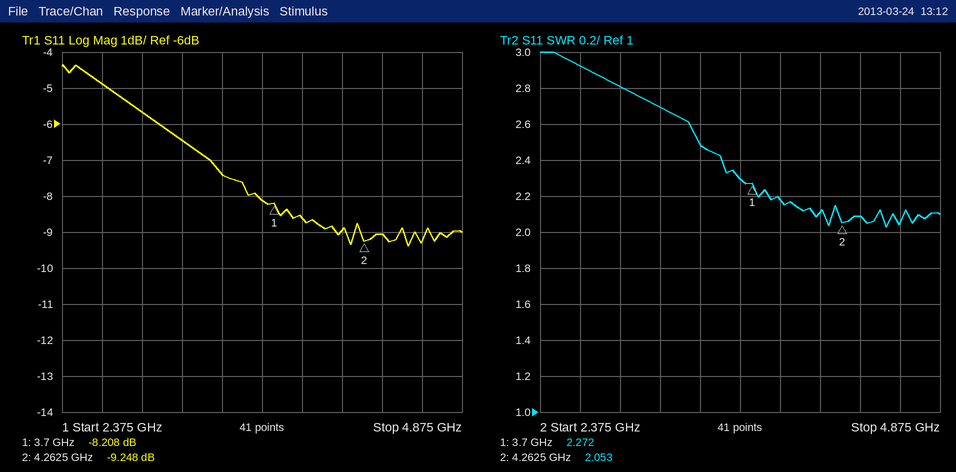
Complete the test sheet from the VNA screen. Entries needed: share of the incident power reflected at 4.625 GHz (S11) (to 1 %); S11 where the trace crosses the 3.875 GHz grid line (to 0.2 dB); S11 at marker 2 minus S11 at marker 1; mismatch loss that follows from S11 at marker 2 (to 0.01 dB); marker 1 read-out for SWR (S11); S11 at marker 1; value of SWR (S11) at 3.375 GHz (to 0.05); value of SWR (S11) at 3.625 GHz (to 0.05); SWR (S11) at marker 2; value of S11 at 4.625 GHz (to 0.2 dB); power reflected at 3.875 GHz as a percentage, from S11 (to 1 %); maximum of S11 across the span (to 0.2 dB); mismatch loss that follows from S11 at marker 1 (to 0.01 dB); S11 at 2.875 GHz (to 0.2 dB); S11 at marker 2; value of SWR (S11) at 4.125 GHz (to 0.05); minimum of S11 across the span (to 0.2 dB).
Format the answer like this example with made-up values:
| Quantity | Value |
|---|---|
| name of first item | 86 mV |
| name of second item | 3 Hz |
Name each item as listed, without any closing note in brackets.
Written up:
| Quantity | Value |
|---|---|
| share of the incident power reflected at 4.625 GHz (S11) | 12 % |
| S11 where the trace crosses the 3.875 GHz grid line | -8.6 dB |
| S11 at marker 2 minus S11 at marker 1 | -1.040 dB |
| mismatch loss that follows from S11 at marker 2 | 0.55 dB |
| marker 1 read-out for SWR | 2.272 |
| S11 at marker 1 | -8.208 dB |
| value of SWR (S11) at 3.375 GHz | 2.50 |
| value of SWR (S11) at 3.625 GHz | 2.30 |
| SWR (S11) at marker 2 | 2.053 |
| value of S11 at 4.625 GHz | -9.2 dB |
| power reflected at 3.875 GHz as a percentage, from S11 | 14 % |
| maximum of S11 across the span | -4.4 dB |
| mismatch loss that follows from S11 at marker 1 | 0.71 dB |
| S11 at 2.875 GHz | -5.6 dB |
| S11 at marker 2 | -9.248 dB |
| value of SWR (S11) at 4.125 GHz | 2.10 |
| minimum of S11 across the span | -9.4 dB |
